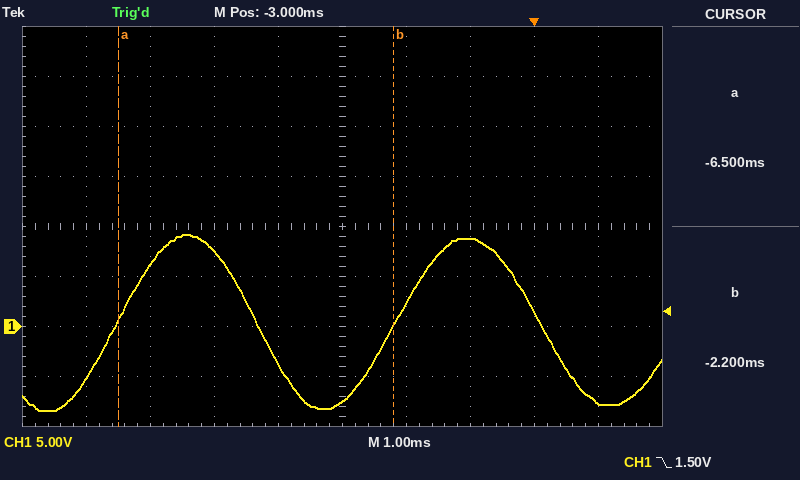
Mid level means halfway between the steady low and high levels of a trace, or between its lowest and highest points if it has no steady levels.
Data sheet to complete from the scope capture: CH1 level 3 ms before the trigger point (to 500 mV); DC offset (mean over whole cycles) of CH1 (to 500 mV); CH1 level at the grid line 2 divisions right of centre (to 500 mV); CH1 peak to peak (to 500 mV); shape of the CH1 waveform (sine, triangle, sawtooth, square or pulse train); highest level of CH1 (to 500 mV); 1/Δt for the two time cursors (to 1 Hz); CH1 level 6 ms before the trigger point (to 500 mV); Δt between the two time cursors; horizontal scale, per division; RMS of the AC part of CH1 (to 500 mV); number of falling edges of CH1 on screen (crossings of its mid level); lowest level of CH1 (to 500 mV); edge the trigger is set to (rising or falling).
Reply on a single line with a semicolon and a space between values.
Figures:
-7.5 V; 500 mV; 9.0 V; 17.5 V; sine; 9.0 V; 233 Hz; 6.0 V; 4.3 ms; 1 ms; 6.0 V; 2; -8.5 V; falling
